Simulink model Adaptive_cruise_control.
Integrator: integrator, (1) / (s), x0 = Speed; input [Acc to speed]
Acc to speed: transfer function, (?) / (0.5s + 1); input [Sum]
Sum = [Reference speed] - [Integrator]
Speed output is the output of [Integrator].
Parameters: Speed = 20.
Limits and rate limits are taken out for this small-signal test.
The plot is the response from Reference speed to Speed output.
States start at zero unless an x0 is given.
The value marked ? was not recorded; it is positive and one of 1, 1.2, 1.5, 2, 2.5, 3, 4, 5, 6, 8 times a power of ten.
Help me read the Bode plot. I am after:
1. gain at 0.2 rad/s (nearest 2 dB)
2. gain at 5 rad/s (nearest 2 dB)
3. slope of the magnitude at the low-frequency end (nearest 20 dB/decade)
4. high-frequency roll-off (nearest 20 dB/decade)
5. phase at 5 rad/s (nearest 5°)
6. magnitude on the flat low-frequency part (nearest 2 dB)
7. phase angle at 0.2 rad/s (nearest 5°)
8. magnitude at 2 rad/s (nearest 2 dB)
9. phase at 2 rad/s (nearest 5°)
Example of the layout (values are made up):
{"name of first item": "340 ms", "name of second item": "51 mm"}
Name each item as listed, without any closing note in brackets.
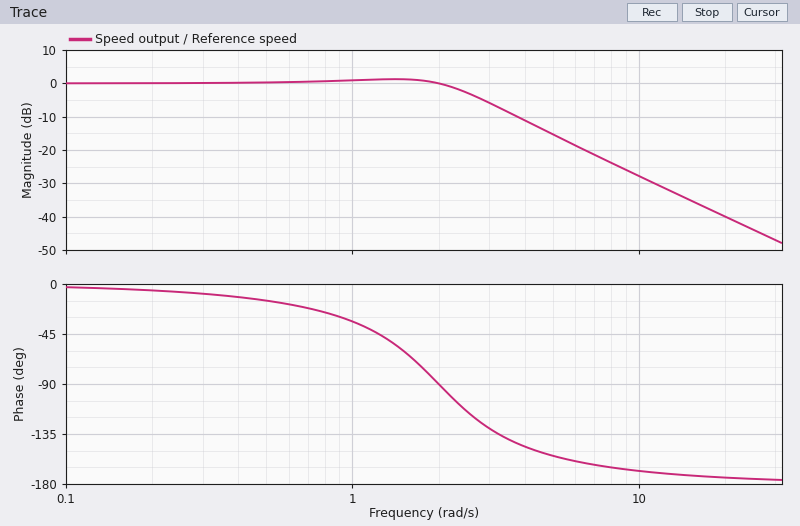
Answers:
{"gain at 0.2 rad/s": "0 dB", "gain at 5 rad/s": "-16 dB", "slope of the magnitude at the low-frequency end": "0 dB/decade", "high-frequency roll-off": "-40 dB/decade", "phase at 5 rad/s": "-155°", "magnitude on the flat low-frequency part": "0 dB", "phase angle at 0.2 rad/s": "-5°", "magnitude at 2 rad/s": "0 dB", "phase at 2 rad/s": "-90°"}
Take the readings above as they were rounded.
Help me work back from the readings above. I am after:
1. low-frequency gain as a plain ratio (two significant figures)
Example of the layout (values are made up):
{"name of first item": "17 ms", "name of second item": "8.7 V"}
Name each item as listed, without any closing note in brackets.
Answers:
{"low-frequency gain as a plain ratio": "1.0"}
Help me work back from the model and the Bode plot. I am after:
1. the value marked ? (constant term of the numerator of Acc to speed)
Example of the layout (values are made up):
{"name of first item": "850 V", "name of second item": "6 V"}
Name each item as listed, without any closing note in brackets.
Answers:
{"the value marked ?": "2"}
